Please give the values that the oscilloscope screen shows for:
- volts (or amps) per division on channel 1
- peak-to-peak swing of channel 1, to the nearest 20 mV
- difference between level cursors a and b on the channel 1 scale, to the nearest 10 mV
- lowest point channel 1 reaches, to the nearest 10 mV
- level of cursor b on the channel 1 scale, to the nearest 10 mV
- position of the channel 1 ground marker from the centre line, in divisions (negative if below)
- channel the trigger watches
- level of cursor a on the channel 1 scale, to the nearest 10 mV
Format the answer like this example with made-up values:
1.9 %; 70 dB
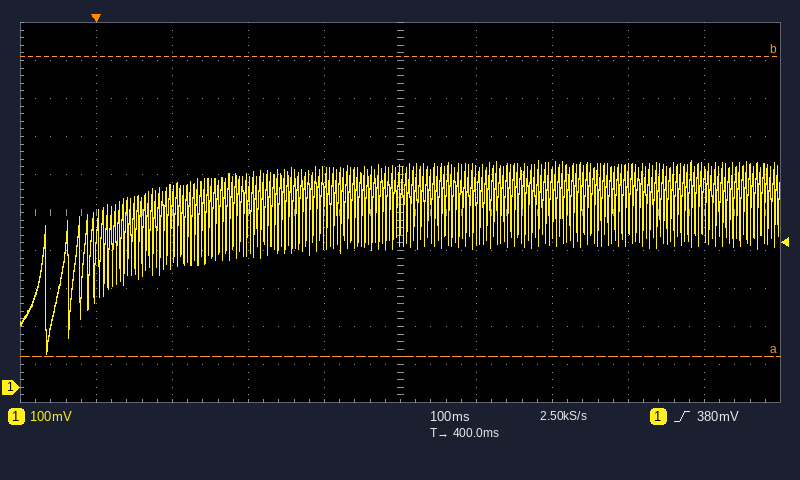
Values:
100 mV; 500 mV; 790 mV; 90 mV; 870 mV; -4.6 div; channel 1; 80 mV
